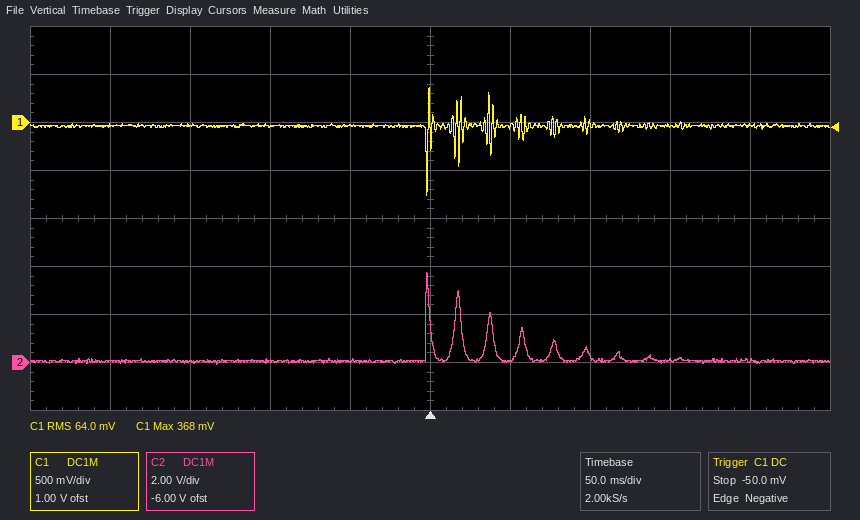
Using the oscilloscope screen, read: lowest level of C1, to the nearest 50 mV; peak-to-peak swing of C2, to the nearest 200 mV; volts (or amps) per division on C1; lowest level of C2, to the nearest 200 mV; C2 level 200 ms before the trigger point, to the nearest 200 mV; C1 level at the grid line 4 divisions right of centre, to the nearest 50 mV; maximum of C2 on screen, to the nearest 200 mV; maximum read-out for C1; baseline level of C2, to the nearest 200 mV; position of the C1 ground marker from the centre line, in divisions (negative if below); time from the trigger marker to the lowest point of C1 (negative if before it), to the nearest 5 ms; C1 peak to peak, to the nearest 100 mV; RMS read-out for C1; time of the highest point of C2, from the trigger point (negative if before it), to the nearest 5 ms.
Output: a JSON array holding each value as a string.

["-750 mV", "3.8 V", "500 mV", "0.0 V", "0.0 V", "-50 mV", "3.8 V", "368 mV", "0.0 V", "+2.0 div", "0 ms", "1.10 V", "64.0 mV", "0 ms"]
